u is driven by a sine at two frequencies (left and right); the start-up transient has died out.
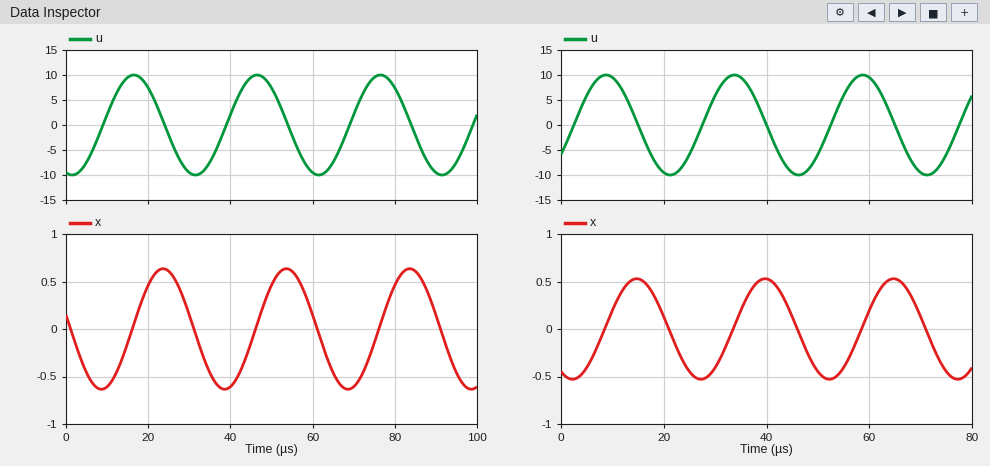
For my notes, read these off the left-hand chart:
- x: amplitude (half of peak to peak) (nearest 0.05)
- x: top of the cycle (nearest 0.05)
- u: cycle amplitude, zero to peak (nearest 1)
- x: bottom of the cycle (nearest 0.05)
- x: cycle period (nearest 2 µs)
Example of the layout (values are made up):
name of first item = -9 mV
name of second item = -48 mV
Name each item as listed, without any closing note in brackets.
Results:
x: amplitude (half of peak to peak) = 0.65
x: top of the cycle = 0.65
u: cycle amplitude, zero to peak = 10
x: bottom of the cycle = -0.65
x: cycle period = 30 µs
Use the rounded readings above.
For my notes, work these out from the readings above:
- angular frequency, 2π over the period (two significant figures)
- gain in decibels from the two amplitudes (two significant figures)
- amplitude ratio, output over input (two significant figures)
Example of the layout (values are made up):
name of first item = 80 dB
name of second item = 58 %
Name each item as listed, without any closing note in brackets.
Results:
angular frequency, 2π over the period = 0.21 rad/µs
gain in decibels from the two amplitudes = -24 dB
amplitude ratio, output over input = 0.065
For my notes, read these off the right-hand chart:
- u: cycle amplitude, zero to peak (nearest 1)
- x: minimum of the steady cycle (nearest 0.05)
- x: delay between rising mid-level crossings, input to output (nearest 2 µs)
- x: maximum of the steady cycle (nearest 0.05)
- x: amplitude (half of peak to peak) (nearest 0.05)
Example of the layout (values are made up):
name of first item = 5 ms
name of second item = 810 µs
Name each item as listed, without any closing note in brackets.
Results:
u: cycle amplitude, zero to peak = 10
x: minimum of the steady cycle = -0.55
x: delay between rising mid-level crossings, input to output = 6 µs
x: maximum of the steady cycle = 0.55
x: amplitude (half of peak to peak) = 0.55
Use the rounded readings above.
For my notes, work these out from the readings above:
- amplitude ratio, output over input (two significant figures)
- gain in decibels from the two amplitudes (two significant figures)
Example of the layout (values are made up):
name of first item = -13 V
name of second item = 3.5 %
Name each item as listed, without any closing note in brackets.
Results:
amplitude ratio, output over input = 0.055
gain in decibels from the two amplitudes = -25 dB
